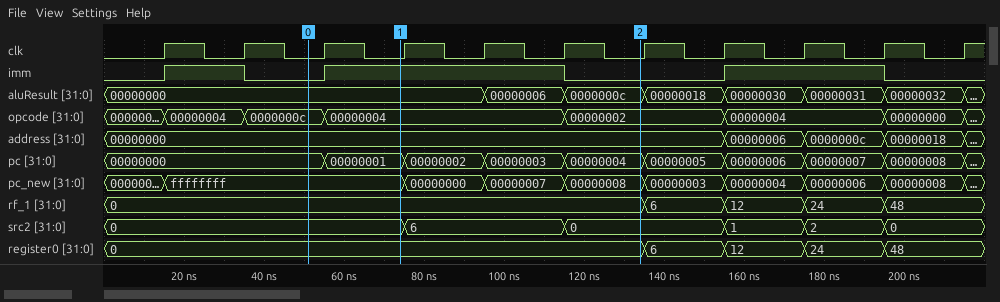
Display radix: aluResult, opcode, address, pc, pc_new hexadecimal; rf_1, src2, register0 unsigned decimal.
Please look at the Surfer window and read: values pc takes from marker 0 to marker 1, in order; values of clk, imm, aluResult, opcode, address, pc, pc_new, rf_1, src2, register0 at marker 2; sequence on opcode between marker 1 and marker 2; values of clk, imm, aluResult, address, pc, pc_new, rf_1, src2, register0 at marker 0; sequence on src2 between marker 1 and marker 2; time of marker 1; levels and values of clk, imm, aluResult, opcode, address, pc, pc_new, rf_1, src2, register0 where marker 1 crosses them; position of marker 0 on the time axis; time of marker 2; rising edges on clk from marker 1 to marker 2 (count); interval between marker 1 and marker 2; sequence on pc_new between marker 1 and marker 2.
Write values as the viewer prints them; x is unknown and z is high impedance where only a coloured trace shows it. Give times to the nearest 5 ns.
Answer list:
00000000, 00000001
clk=0, imm=0, aluResult=0000000c, opcode=00000002, address=00000000, pc=00000004, pc_new=00000008, rf_1=0, src2=0, register0=0
00000004, 00000002
clk=0, imm=0, aluResult=00000000, address=00000000, pc=00000000, pc_new=ffffffff, rf_1=0, src2=0, register0=0
0, 6, 0
75 ns
clk=0, imm=1, aluResult=00000000, opcode=00000004, address=00000000, pc=00000001, pc_new=ffffffff, rf_1=0, src2=0, register0=0
50 ns
135 ns
3
60 ns
ffffffff, 00000000, 00000007, 00000008
